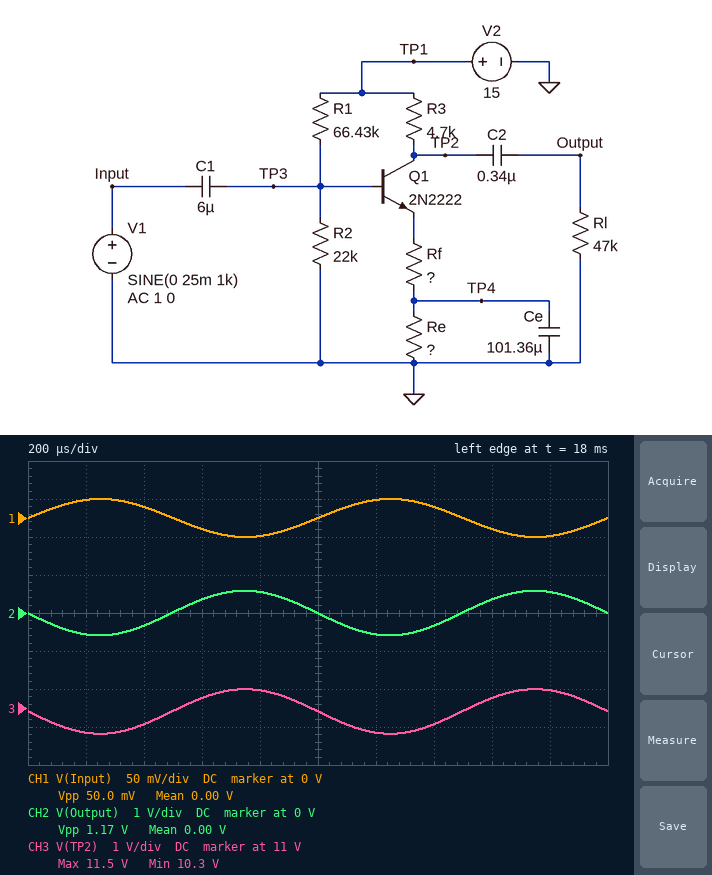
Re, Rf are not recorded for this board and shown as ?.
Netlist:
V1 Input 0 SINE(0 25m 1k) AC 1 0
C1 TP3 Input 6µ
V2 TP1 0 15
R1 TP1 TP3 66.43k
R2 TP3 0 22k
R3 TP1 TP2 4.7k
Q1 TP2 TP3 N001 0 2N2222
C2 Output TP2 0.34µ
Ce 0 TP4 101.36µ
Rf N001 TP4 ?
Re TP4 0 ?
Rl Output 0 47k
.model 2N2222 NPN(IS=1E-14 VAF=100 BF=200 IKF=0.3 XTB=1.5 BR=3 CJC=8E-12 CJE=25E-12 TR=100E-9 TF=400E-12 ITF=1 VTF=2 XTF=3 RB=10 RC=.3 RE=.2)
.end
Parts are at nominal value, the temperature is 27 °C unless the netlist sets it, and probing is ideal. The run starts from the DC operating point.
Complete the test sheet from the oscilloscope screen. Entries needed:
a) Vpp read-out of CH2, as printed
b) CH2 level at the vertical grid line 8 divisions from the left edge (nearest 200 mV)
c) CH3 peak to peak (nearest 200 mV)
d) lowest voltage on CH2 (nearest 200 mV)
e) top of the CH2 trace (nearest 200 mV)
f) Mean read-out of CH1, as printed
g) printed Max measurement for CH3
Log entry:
1.17 V
400 mV
1.2 V
-600 mV
600 mV
0.00 V
11.5 V
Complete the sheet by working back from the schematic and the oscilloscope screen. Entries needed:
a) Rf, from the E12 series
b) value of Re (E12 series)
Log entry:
150 Ω
3.3 kΩ
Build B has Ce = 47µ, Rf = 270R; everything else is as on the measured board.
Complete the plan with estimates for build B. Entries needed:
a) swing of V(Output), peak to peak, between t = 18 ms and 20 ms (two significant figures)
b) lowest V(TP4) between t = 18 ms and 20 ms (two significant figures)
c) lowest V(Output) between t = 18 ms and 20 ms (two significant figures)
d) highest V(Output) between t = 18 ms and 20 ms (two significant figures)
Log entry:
700 mV
2.8 V
-350 mV
350 mV
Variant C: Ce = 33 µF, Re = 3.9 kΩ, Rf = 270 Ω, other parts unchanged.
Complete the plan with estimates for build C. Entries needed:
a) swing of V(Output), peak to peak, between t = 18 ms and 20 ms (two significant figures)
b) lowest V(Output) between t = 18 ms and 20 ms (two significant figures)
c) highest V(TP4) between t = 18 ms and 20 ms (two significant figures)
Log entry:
690 mV
-350 mV
2.8 V
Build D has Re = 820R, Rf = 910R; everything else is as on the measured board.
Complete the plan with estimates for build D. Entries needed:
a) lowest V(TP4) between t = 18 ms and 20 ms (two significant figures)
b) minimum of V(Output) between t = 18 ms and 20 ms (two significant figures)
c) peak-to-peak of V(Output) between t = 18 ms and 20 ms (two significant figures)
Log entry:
1.4 V
-110 mV
230 mV
